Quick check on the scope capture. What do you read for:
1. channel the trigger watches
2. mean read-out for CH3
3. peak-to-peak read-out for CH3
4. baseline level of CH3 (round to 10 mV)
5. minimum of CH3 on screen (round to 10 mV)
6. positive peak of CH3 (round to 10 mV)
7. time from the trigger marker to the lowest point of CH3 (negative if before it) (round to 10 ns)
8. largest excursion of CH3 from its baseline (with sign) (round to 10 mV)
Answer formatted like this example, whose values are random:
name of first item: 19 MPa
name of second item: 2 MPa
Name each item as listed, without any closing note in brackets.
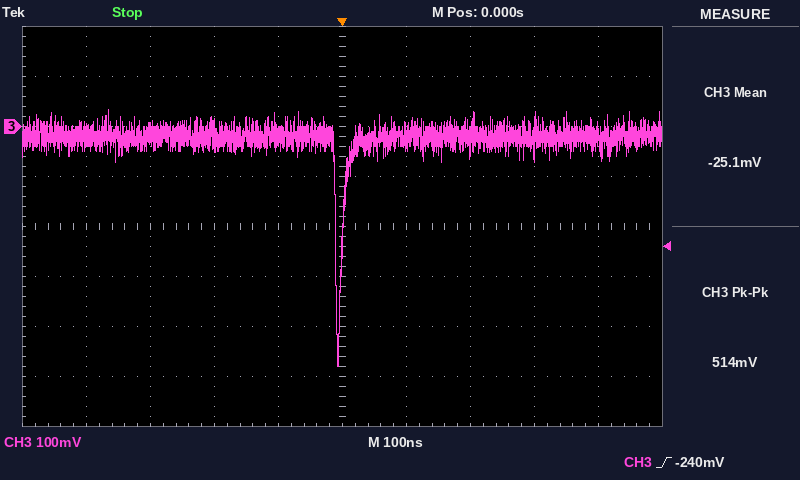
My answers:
channel the trigger watches: CH3
mean read-out for CH3: -25.1 mV
peak-to-peak read-out for CH3: 514 mV
baseline level of CH3: -20 mV
minimum of CH3 on screen: -480 mV
positive peak of CH3: 30 mV
time from the trigger marker to the lowest point of CH3 (negative if before it): -10 ns
largest excursion of CH3 from its baseline (with sign): -460 mV
